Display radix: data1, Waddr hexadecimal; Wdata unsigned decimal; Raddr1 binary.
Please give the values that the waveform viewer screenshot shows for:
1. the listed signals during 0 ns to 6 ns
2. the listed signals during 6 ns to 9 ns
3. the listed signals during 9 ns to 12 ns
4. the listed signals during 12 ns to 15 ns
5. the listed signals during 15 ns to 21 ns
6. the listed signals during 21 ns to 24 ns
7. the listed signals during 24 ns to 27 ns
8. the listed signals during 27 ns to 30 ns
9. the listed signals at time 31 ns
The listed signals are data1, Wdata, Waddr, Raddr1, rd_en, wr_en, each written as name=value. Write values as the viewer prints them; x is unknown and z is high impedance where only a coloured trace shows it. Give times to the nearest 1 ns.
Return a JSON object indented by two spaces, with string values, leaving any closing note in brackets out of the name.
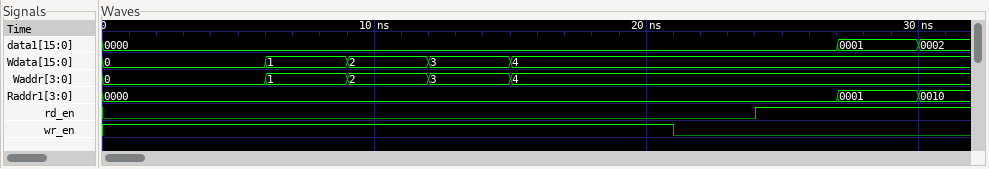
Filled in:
{
  "the listed signals during 0 ns to 6 ns": "data1=0000, Wdata=0, Waddr=0, Raddr1=0000, rd_en=0, wr_en=1",
  "the listed signals during 6 ns to 9 ns": "data1=0000, Wdata=1, Waddr=1, Raddr1=0000, rd_en=0, wr_en=1",
  "the listed signals during 9 ns to 12 ns": "data1=0000, Wdata=2, Waddr=2, Raddr1=0000, rd_en=0, wr_en=1",
  "the listed signals during 12 ns to 15 ns": "data1=0000, Wdata=3, Waddr=3, Raddr1=0000, rd_en=0, wr_en=1",
  "the listed signals during 15 ns to 21 ns": "data1=0000, Wdata=4, Waddr=4, Raddr1=0000, rd_en=0, wr_en=1",
  "the listed signals during 21 ns to 24 ns": "data1=0000, Wdata=4, Waddr=4, Raddr1=0000, rd_en=0, wr_en=0",
  "the listed signals during 24 ns to 27 ns": "data1=0000, Wdata=4, Waddr=4, Raddr1=0000, rd_en=1, wr_en=0",
  "the listed signals during 27 ns to 30 ns": "data1=0001, Wdata=4, Waddr=4, Raddr1=0001, rd_en=1, wr_en=0",
  "the listed signals at time 31 ns": "data1=0002, Wdata=4, Waddr=4, Raddr1=0010, rd_en=1, wr_en=0"
}
